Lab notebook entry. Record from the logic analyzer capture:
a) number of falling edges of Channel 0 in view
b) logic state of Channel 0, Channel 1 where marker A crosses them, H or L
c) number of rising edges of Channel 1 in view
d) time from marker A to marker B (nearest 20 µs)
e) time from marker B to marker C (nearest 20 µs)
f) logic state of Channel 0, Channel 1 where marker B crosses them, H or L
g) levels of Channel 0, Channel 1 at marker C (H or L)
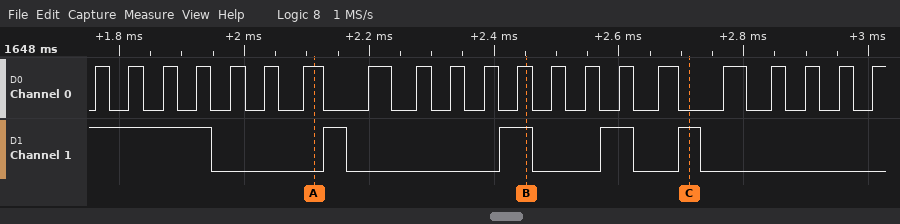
20
Channel 0=H, Channel 1=L
4
340 µs
260 µs
Channel 0=H, Channel 1=H
Channel 0=L, Channel 1=H
